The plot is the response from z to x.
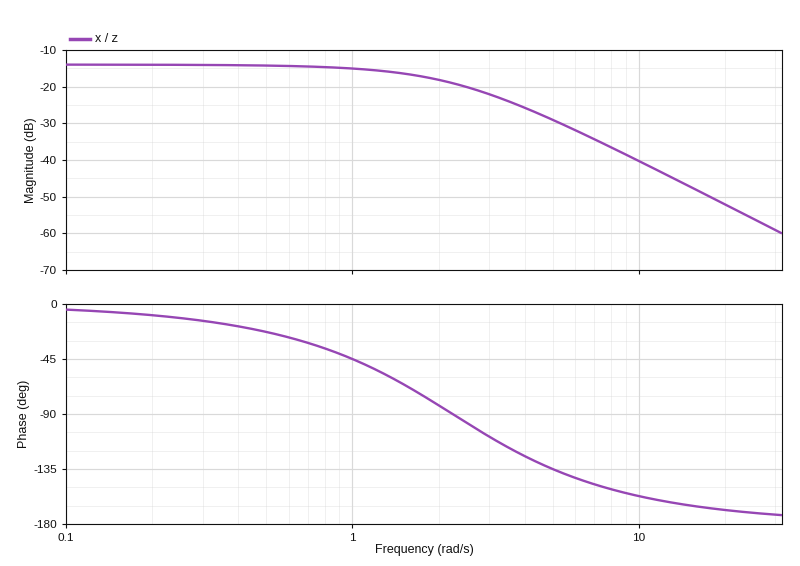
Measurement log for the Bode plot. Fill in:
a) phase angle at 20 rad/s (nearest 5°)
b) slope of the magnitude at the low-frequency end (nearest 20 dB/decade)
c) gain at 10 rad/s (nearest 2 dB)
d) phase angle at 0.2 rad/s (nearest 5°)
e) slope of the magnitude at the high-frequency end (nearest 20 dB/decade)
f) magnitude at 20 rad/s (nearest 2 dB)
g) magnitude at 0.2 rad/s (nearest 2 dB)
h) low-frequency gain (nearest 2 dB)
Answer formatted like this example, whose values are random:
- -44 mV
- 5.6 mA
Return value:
- -170°
- 0 dB/decade
- -40 dB
- -10°
- -40 dB/decade
- -52 dB
- -14 dB
- -14 dB
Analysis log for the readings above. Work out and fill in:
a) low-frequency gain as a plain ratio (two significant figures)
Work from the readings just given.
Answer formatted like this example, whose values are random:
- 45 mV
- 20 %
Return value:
- 0.20
